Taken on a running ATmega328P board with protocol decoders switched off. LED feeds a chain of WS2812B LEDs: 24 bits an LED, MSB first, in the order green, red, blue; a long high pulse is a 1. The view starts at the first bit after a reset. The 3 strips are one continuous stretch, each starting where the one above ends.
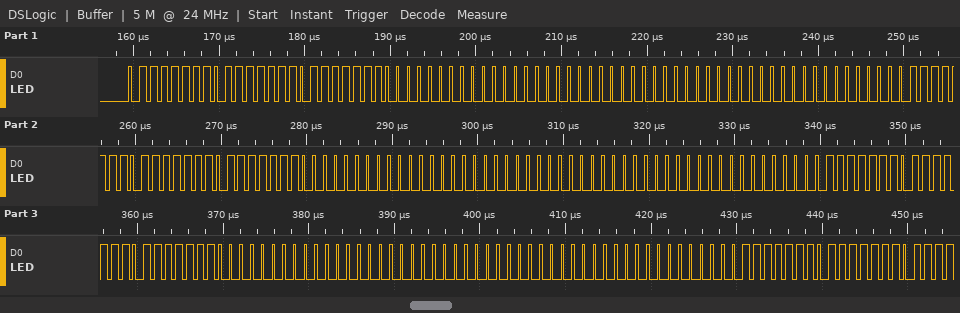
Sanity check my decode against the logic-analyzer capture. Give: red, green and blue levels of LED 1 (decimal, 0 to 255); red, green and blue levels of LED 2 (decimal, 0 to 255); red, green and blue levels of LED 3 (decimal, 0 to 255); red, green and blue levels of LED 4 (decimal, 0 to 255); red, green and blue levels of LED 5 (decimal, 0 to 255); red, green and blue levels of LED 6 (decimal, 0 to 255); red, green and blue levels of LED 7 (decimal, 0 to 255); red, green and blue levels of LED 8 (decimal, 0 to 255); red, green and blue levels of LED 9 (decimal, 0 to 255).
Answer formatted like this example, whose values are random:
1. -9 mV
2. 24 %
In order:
1. 127, 127, 127
2. 0, 0, 0
3. 0, 0, 0
4. 127, 127, 127
5. 0, 0, 0
6. 0, 0, 0
7. 127, 127, 127
8. 0, 0, 0
9. 0, 0, 0
